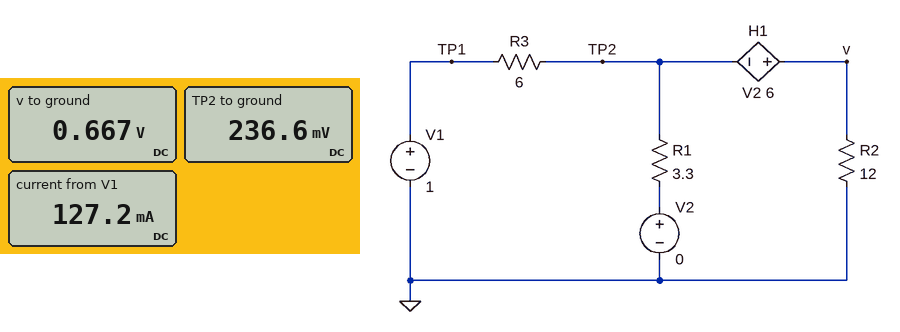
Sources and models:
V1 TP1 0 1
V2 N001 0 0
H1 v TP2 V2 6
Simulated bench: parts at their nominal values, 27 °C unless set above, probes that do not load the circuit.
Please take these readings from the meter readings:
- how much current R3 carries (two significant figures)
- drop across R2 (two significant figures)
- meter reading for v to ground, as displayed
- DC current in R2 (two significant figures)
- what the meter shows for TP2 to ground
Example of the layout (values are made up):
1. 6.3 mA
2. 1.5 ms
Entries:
1. 130 mA
2. 670 mV
3. 0.667 V
4. 56 mA
5. 236.6 mV
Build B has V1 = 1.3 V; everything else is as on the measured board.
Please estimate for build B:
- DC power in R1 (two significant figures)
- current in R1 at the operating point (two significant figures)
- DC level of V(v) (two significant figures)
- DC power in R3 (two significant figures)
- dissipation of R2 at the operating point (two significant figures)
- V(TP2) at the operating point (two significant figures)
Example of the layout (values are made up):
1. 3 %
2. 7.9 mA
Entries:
1. 29 mW
2. 93 mA
3. 870 mV
4. 160 mW
5. 63 mW
6. 310 mV
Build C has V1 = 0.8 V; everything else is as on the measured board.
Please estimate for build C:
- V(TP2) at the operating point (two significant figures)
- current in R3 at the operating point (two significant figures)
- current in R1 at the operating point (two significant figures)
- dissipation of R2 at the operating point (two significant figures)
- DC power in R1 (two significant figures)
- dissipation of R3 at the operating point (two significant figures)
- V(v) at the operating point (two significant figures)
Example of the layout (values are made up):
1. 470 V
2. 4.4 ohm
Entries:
1. 190 mV
2. 100 mA
3. 57 mA
4. 24 mW
5. 11 mW
6. 62 mW
7. 530 mV
